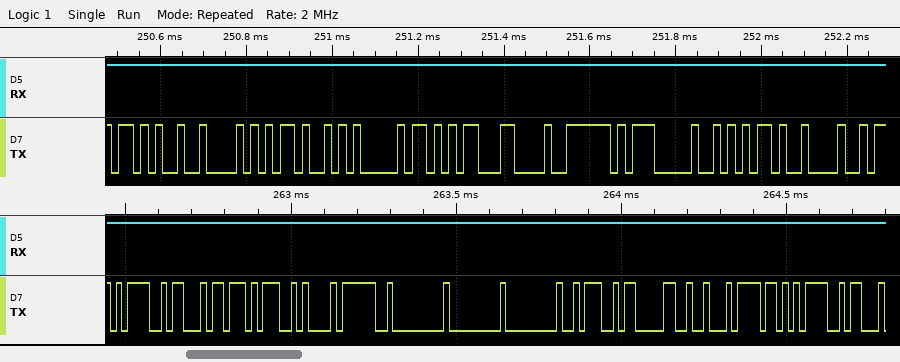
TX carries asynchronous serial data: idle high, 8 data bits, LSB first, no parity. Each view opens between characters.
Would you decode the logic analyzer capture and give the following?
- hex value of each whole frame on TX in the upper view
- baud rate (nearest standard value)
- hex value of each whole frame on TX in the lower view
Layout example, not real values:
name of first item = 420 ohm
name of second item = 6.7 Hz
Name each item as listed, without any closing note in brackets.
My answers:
hex value of each whole frame on TX in the upper view = 2B, 42, 2D, 05, AB, 0C, 7E, 07, AA, 09
baud rate = 57600 baud
hex value of each whole frame on TX in the lower view = 3D, A3, D7, 0A, 3F, 00, 00, 00, 3A, 83, 12, 6F, 3D
